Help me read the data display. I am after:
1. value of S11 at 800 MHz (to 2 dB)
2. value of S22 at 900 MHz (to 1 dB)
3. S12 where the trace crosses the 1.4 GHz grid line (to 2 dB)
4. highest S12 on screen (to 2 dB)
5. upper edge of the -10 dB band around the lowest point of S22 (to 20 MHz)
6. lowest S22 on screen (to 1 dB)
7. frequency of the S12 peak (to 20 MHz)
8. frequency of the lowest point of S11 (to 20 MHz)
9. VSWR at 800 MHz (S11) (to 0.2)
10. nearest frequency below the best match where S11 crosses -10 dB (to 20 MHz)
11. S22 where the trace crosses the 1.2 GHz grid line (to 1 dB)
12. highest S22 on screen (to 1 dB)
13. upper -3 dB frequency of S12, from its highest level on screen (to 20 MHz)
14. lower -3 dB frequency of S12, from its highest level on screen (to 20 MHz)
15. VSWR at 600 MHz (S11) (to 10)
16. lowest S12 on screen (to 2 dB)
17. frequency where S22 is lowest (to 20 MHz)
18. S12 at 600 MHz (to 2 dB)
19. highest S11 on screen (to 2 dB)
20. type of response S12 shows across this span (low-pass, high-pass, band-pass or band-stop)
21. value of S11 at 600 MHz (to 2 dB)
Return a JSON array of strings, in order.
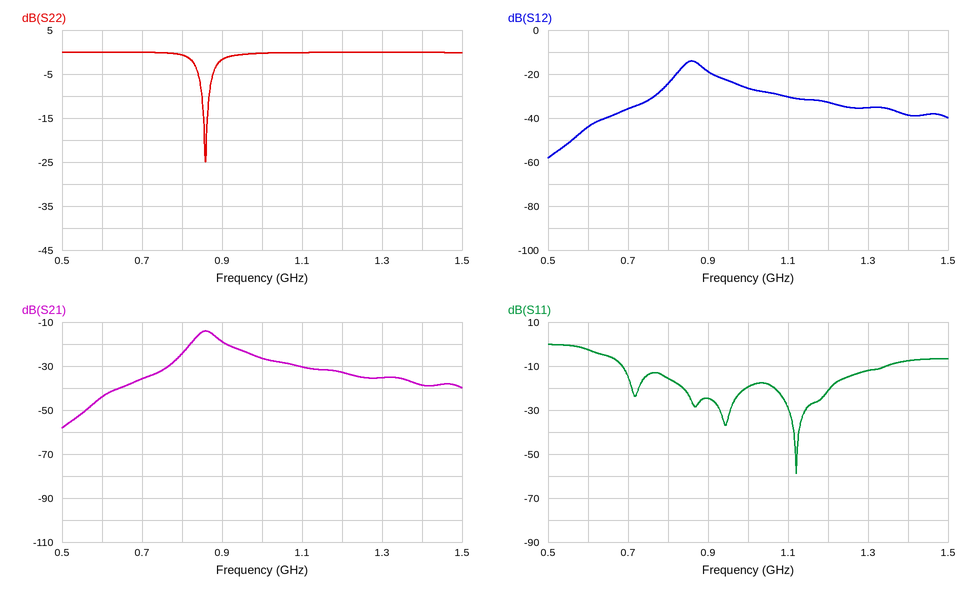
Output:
["-16 dB", "-2 dB", "-38 dB", "-14 dB", "860 MHz", "-25 dB", "860 MHz", "1.12 GHz", "1.4", "680 MHz", "0 dB", "0 dB", "880 MHz", "840 MHz", "10", "-58 dB", "860 MHz", "-44 dB", "0 dB", "band-pass", "-2 dB"]
